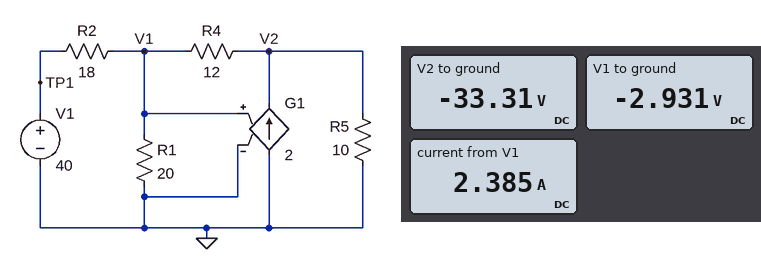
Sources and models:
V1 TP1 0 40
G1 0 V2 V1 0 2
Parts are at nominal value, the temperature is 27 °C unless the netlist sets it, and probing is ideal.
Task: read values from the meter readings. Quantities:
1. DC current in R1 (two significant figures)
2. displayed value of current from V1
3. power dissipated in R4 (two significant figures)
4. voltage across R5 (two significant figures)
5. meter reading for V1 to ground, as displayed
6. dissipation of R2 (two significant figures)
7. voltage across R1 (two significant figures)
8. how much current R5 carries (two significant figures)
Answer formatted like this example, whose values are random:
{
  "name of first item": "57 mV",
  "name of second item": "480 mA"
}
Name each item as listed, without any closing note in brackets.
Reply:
{
  "DC current in R1": "150 mA",
  "displayed value of current from V1": "2.385 A",
  "power dissipated in R4": "77 W",
  "voltage across R5": "33 V",
  "meter reading for V1 to ground, as displayed": "-2.931 V",
  "dissipation of R2": "100 W",
  "voltage across R1": "2.9 V",
  "how much current R5 carries": "3.3 A"
}
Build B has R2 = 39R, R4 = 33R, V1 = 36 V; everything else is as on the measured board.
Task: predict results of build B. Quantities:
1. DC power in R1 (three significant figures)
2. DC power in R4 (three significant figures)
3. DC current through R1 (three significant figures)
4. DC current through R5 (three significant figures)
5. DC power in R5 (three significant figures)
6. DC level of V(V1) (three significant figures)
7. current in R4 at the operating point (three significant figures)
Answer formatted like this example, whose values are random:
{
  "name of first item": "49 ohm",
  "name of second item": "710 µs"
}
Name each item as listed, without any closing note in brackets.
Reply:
{
  "DC power in R1": "318 mW",
  "DC power in R4": "40.9 W",
  "DC current through R1": "126 mA",
  "DC current through R5": "3.93 A",
  "DC power in R5": "154 W",
  "DC level of V(V1)": "-2.52 V",
  "current in R4 at the operating point": "1.11 A"
}
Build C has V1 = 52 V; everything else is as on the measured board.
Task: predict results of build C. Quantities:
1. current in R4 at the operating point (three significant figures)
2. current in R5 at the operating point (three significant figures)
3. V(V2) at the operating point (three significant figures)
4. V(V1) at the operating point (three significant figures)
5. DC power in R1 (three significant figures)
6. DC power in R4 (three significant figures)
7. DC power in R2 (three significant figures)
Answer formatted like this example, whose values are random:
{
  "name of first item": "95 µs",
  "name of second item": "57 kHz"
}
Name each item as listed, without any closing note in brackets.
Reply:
{
  "current in R4 at the operating point": "3.29 A",
  "current in R5 at the operating point": "4.33 A",
  "V(V2) at the operating point": "-43.3 V",
  "V(V1) at the operating point": "-3.81 V",
  "DC power in R1": "726 mW",
  "DC power in R4": "130 W",
  "DC power in R2": "173 W"
}
